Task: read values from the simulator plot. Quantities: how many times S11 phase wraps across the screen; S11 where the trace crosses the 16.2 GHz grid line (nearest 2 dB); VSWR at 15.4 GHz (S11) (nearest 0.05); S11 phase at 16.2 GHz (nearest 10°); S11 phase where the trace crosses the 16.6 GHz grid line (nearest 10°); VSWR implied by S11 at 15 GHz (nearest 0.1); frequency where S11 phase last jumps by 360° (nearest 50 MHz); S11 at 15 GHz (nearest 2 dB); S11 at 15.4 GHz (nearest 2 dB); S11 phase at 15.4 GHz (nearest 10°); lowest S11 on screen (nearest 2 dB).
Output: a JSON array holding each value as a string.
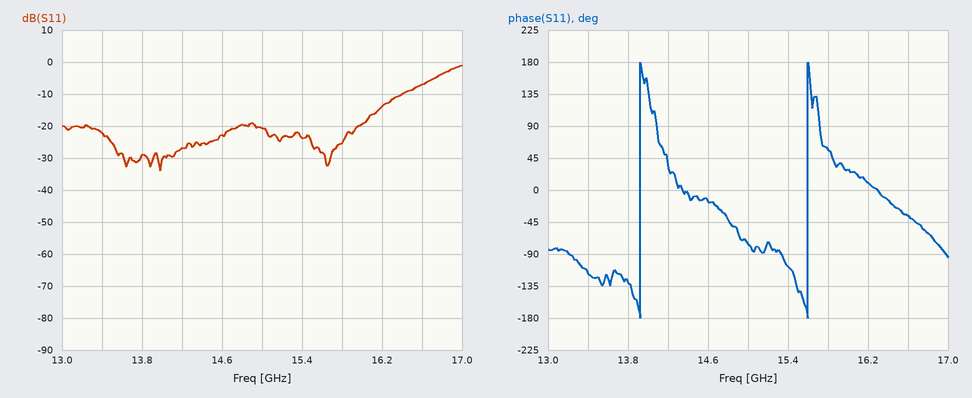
["2", "-14 dB", "1.15", "10°", "-40°", "1.2", "15.60 GHz", "-20 dB", "-24 dB", "-110°", "-34 dB"]
